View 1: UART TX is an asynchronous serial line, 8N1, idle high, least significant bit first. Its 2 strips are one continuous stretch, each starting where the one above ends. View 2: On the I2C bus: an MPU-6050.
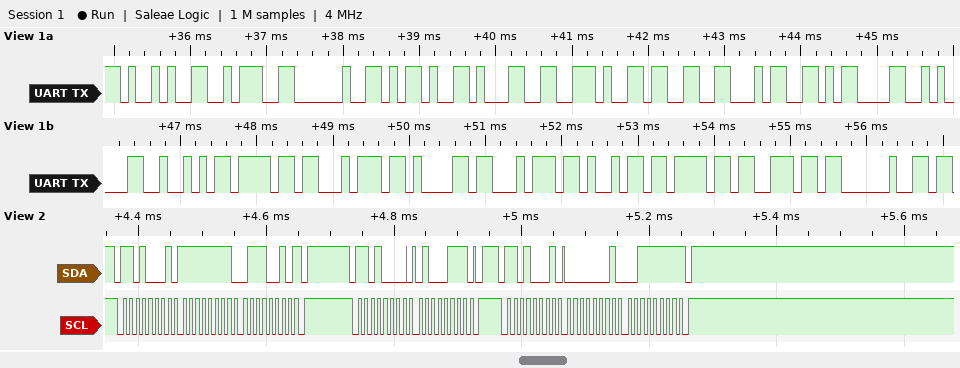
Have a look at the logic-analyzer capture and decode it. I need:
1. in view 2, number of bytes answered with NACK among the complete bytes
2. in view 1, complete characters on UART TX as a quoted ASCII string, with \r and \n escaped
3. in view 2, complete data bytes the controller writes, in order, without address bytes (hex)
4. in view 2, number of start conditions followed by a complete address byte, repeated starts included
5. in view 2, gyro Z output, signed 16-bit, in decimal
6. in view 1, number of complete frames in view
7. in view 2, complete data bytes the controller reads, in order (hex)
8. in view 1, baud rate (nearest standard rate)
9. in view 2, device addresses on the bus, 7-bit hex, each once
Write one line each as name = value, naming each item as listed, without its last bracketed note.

in view 2, number of bytes answered with NACK among the complete bytes = 2
in view 1, complete characters on UART TX as a quoted ASCII string, with \r and \n escaped = "): -1.34\r\nRotation "
in view 2, complete data bytes the controller writes, in order, without address bytes = 47
in view 2, number of start conditions followed by a complete address byte, repeated starts included = 3
in view 2, gyro Z output, signed 16-bit, in decimal = 319
in view 1, number of complete frames in view = 19
in view 2, complete data bytes the controller reads, in order = FF 72 01 3F
in view 1, baud rate = 9600 baud
in view 2, device addresses on the bus, 7-bit hex, each once = 0x68
